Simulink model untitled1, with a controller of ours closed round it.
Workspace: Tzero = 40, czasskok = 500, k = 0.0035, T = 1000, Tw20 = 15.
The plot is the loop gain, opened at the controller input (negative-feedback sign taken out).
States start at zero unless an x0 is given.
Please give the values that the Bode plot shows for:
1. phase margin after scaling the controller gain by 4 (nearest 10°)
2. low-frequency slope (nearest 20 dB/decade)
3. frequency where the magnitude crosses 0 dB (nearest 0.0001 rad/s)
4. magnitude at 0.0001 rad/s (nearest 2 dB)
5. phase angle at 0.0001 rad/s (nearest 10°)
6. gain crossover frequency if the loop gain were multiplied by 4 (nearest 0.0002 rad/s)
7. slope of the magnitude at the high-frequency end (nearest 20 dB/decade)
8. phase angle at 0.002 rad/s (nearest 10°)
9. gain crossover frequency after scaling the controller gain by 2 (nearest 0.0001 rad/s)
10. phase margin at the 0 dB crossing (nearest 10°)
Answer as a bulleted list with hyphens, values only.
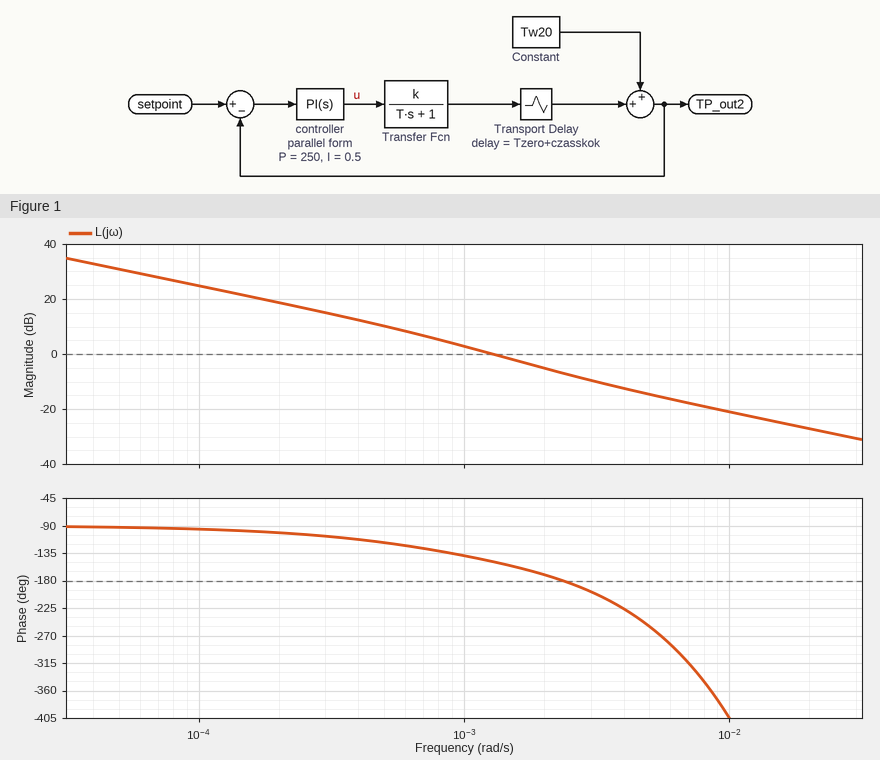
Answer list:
- -40°
- -20 dB/decade
- 0.0013 rad/s
- 24 dB
- -100°
- 0.0038 rad/s
- -20 dB/decade
- -170°
- 0.0022 rad/s
- 30°
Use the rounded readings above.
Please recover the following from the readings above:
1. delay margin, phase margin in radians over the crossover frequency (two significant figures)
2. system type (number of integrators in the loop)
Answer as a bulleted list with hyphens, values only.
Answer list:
- 400 s
- 1
